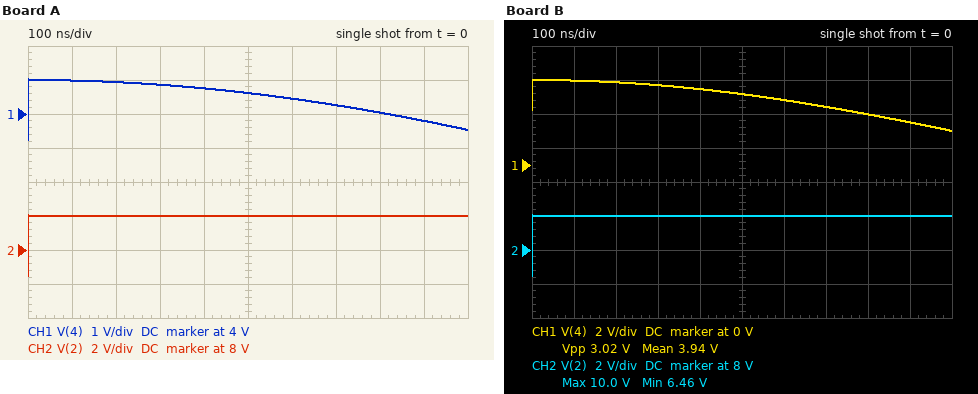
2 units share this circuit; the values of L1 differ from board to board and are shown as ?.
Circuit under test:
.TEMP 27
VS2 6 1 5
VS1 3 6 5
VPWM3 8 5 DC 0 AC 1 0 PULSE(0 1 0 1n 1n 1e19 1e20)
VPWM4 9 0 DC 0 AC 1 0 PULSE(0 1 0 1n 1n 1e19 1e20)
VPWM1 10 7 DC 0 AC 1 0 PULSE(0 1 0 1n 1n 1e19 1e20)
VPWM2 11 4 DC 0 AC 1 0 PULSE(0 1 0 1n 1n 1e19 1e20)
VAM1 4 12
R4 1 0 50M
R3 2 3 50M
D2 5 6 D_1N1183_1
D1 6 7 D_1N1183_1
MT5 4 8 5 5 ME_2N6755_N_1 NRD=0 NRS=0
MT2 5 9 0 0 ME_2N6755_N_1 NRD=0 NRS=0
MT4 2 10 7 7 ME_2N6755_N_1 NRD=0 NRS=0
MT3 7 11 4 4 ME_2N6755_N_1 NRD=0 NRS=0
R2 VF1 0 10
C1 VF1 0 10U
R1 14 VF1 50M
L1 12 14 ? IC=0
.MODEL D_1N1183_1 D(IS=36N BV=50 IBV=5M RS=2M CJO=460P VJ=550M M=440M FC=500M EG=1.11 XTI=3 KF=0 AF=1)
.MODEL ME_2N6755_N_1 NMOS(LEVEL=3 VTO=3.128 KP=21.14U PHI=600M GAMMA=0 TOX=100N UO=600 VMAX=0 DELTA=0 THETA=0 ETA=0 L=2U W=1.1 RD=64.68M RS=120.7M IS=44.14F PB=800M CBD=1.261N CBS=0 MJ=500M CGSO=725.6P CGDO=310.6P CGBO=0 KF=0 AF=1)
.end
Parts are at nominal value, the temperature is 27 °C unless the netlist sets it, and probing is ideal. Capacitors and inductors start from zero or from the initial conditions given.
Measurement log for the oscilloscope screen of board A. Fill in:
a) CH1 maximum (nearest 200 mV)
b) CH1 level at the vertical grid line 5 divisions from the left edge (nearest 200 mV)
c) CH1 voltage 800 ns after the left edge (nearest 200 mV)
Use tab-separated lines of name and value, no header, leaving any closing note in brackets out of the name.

CH1 maximum	5.0 V
CH1 level at the vertical grid line 5 divisions from the left edge	4.6 V
CH1 voltage 800 ns after the left edge	4.0 V
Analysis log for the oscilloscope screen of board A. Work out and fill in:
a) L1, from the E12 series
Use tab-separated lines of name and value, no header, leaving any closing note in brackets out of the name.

L1, from the E12 series	1.5 mH
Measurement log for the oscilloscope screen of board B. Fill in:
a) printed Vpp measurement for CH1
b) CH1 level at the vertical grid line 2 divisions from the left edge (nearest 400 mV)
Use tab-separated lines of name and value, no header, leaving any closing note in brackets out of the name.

printed Vpp measurement for CH1	3.02 V
CH1 level at the vertical grid line 2 divisions from the left edge	4.8 V
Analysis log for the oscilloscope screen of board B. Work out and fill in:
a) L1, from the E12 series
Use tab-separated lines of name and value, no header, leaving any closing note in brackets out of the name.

L1, from the E12 series	680 µH
